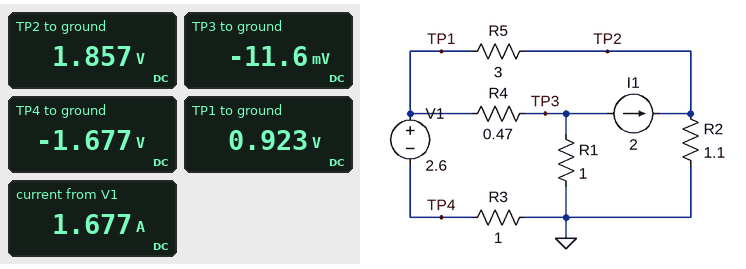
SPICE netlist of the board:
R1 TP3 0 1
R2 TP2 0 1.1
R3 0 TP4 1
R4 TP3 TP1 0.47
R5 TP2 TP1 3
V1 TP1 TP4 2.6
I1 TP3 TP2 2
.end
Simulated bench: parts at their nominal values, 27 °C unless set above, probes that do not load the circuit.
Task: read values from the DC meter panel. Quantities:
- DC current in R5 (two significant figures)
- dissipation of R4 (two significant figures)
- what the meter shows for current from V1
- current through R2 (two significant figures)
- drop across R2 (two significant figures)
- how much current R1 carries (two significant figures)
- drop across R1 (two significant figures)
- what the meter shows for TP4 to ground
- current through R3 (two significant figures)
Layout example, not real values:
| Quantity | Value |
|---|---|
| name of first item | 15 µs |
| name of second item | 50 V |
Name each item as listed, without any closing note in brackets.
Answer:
| Quantity | Value |
|---|---|
| DC current in R5 | 310 mA |
| dissipation of R4 | 1.9 W |
| what the meter shows for current from V1 | 1.677 A |
| current through R2 | 1.7 A |
| drop across R2 | 1.9 V |
| how much current R1 carries | 12 mA |
| drop across R1 | 12 mV |
| what the meter shows for TP4 to ground | -1.677 V |
| current through R3 | 1.7 A |
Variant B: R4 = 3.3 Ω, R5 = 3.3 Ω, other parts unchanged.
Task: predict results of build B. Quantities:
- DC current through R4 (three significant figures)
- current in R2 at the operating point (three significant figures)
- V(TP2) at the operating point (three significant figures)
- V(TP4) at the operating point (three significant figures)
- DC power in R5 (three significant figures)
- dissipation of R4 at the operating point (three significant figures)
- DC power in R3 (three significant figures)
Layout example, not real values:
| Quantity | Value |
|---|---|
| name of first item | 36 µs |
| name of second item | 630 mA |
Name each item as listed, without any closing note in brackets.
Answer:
| Quantity | Value |
|---|---|
| DC current through R4 | 885 mA |
| current in R2 at the operating point | 1.91 A |
| V(TP2) at the operating point | 2.10 V |
| V(TP4) at the operating point | -795 mV |
| DC power in R5 | 26.6 mW |
| dissipation of R4 at the operating point | 2.58 W |
| DC power in R3 | 632 mW |
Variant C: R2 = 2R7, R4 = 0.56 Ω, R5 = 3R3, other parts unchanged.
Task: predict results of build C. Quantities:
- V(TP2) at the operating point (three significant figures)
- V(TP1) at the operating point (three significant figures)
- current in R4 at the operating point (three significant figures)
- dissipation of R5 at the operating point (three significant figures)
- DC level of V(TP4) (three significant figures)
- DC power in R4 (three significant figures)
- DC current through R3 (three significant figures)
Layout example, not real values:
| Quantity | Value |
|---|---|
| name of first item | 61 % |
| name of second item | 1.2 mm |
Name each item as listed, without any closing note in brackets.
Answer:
| Quantity | Value |
|---|---|
| V(TP2) at the operating point | 3.52 V |
| V(TP1) at the operating point | 1.23 V |
| current in R4 at the operating point | 2.07 A |
| dissipation of R5 at the operating point | 1.60 W |
| DC level of V(TP4) | -1.37 V |
| DC power in R4 | 2.40 W |
| DC current through R3 | 1.37 A |
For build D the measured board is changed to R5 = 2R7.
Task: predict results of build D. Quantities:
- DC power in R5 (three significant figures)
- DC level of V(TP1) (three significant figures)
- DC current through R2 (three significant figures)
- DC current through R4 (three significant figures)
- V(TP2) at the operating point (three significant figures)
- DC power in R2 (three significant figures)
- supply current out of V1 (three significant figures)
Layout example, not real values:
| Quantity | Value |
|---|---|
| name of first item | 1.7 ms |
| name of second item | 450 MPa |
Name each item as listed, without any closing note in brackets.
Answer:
| Quantity | Value |
|---|---|
| DC power in R5 | 299 mW |
| DC level of V(TP1) | 936 mV |
| DC current through R2 | 1.67 A |
| DC current through R4 | 2.00 A |
| V(TP2) at the operating point | 1.83 V |
| DC power in R2 | 3.06 W |
| supply current out of V1 | 1.66 A |
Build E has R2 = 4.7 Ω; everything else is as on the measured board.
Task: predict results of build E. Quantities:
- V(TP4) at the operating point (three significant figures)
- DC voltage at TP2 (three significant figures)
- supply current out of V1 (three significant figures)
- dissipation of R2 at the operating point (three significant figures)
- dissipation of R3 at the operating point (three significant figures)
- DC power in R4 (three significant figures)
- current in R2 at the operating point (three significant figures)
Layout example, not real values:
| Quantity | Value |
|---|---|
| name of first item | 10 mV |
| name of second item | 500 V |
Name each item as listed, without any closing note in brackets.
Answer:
| Quantity | Value |
|---|---|
| V(TP4) at the operating point | -1.24 V |
| DC voltage at TP2 | 4.49 V |
| supply current out of V1 | 1.24 A |
| dissipation of R2 at the operating point | 4.29 W |
| dissipation of R3 at the operating point | 1.54 W |
| DC power in R4 | 2.45 W |
| current in R2 at the operating point | 956 mA |
